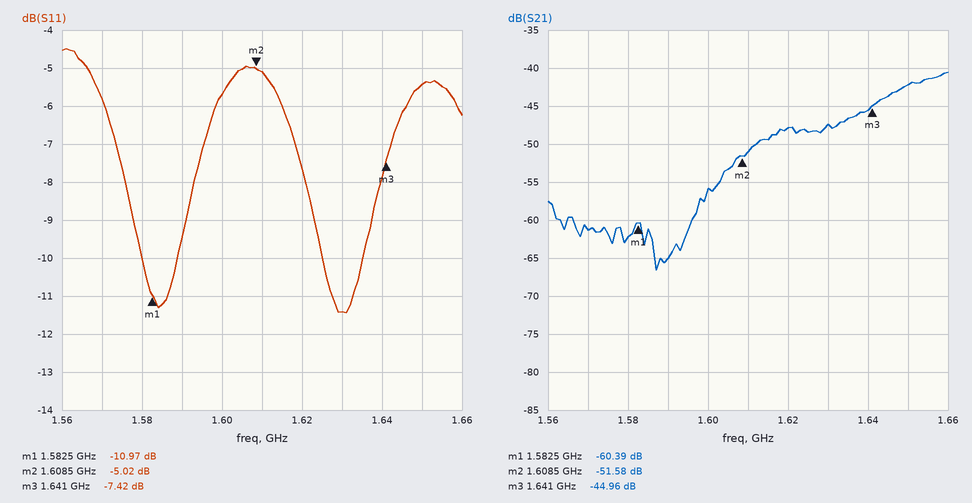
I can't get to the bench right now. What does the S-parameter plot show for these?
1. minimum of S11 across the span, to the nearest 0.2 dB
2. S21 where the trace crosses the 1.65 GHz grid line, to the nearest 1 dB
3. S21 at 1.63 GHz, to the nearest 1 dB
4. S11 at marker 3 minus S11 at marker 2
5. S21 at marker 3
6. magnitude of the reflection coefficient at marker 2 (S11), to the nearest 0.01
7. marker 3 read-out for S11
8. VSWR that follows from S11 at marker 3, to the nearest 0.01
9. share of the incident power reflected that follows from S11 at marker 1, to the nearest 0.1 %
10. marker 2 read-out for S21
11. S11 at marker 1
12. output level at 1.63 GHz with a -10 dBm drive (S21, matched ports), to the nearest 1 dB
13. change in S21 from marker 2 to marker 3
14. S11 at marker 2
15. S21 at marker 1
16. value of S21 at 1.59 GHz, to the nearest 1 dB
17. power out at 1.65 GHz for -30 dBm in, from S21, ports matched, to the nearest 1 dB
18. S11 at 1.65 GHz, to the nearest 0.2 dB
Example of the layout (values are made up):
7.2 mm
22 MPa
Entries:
-11.4 dB
-42 dB
-47 dB
-2.40 dB
-44.96 dB
0.56
-7.42 dB
2.48
8.0 %
-51.58 dB
-10.97 dB
-57 dBm
6.62 dB
-5.02 dB
-60.39 dB
-65 dB
-72 dBm
-5.4 dB
